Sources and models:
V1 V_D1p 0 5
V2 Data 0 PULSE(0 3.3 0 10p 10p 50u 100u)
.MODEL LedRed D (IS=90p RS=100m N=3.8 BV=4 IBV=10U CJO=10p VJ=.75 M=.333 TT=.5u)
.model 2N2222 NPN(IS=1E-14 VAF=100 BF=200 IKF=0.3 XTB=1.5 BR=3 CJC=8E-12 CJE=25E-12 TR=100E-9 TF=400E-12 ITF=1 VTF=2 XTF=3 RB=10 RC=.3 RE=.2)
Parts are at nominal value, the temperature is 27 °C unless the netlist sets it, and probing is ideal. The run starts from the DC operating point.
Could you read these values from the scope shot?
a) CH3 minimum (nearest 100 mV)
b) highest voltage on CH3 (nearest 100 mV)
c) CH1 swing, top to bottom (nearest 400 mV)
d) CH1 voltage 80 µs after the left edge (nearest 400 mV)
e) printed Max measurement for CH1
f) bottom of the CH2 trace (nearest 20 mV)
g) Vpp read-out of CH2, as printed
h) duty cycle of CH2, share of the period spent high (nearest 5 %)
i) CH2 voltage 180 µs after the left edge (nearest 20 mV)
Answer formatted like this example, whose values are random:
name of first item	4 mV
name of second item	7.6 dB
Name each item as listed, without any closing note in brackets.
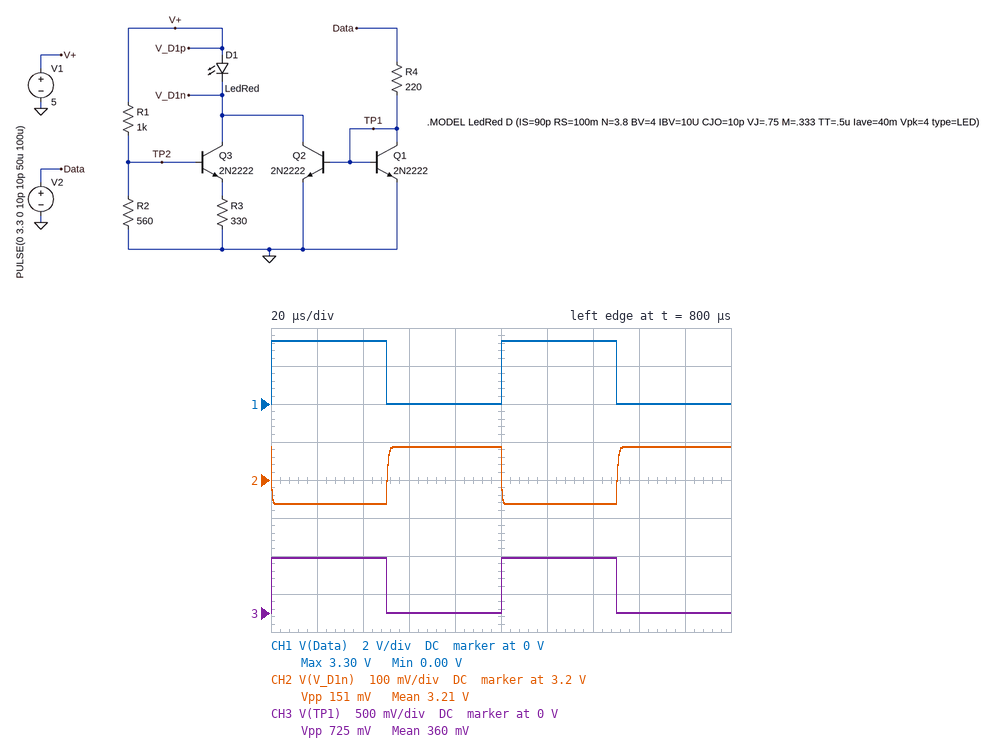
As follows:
CH3 minimum	0 V
highest voltage on CH3	700 mV
CH1 swing, top to bottom	3.2 V
CH1 voltage 80 µs after the left edge	0 V
printed Max measurement for CH1	3.30 V
bottom of the CH2 trace	3.14 V
Vpp read-out of CH2, as printed	151 mV
duty cycle of CH2, share of the period spent high	50 %
CH2 voltage 180 µs after the left edge	3.28 V
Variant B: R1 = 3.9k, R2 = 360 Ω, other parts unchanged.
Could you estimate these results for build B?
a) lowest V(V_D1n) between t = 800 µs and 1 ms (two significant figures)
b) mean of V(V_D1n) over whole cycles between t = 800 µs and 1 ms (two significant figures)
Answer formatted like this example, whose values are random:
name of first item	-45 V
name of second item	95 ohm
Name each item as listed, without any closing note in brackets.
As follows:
lowest V(V_D1n) between t = 800 µs and 1 ms	3.2 V
mean of V(V_D1n) over whole cycles between t = 800 µs and 1 ms	3.7 V
